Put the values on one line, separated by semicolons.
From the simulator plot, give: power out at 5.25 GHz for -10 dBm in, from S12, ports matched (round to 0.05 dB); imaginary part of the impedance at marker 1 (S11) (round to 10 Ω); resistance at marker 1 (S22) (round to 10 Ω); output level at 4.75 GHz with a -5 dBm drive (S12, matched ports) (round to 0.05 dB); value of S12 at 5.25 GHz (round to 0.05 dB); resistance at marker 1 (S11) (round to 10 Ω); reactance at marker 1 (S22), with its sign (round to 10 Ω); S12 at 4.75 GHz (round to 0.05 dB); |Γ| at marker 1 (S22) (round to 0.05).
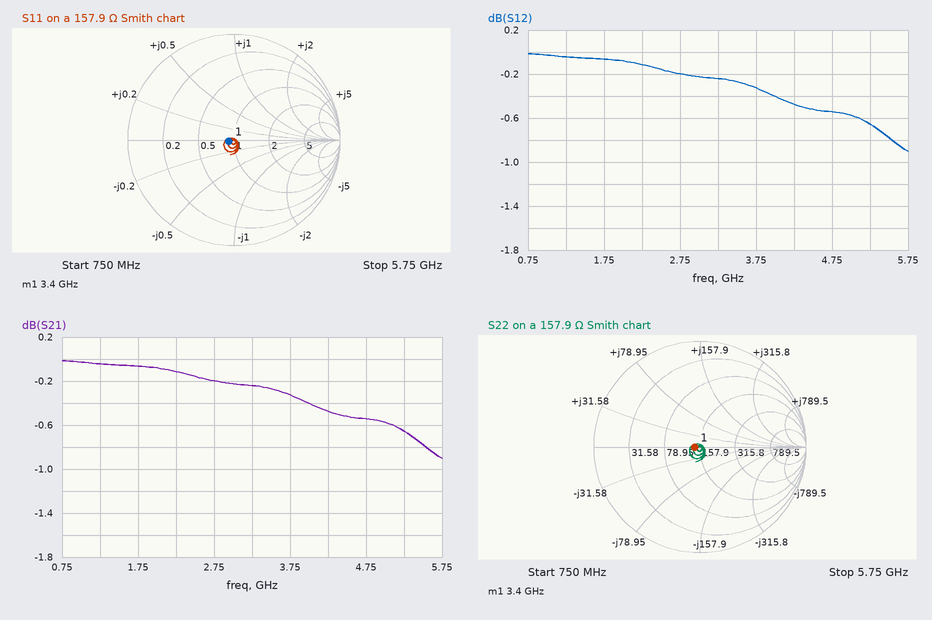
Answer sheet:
-10.65 dBm; 0 Ω; 140 Ω; -5.55 dBm; -0.65 dB; 140 Ω; 0 Ω; -0.55 dB; 0.05
